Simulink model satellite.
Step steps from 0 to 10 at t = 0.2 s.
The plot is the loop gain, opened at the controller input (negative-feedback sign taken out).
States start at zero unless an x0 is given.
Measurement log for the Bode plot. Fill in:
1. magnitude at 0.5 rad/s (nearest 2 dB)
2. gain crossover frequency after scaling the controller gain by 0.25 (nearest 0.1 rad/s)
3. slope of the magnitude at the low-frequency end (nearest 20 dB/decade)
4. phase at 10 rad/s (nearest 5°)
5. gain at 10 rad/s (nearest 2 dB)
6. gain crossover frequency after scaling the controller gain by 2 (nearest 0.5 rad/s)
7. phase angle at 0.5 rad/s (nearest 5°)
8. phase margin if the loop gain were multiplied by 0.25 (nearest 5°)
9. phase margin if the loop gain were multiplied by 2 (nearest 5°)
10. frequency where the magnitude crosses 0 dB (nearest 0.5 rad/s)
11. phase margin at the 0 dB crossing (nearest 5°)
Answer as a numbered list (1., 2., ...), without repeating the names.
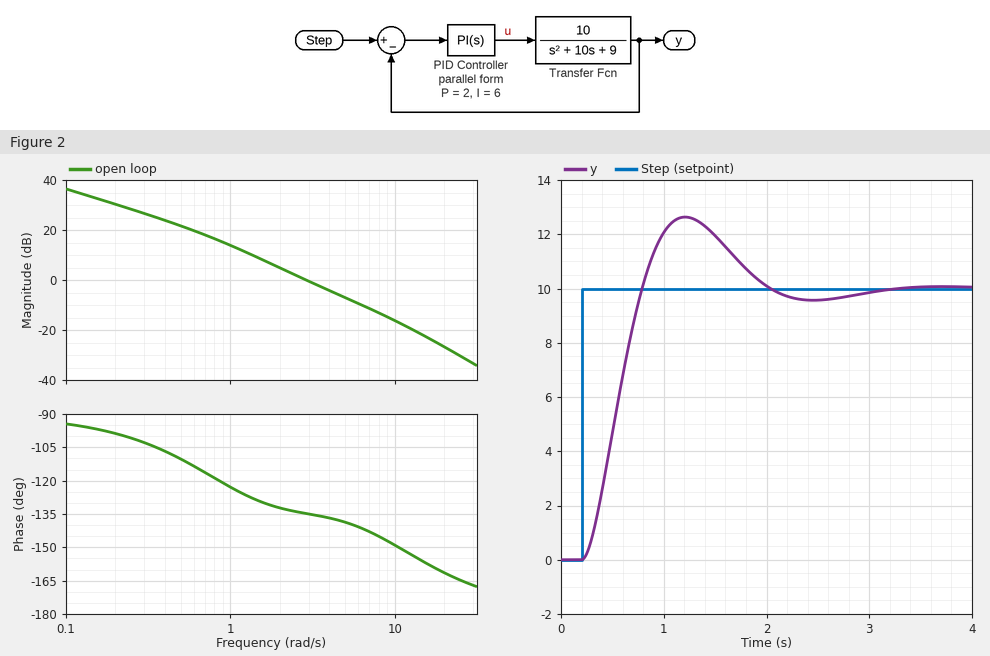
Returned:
1. 22 dB
2. 1.2 rad/s
3. -20 dB/decade
4. -150°
5. -16 dB
6. 4.5 rad/s
7. -110°
8. 55°
9. 40°
10. 3.0 rad/s
11. 45°
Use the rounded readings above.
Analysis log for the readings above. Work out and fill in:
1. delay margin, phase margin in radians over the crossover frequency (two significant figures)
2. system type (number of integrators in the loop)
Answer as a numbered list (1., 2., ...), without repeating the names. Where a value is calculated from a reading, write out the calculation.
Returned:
1. 45 × π / 180 / 3 = 0.26 s
2. 1
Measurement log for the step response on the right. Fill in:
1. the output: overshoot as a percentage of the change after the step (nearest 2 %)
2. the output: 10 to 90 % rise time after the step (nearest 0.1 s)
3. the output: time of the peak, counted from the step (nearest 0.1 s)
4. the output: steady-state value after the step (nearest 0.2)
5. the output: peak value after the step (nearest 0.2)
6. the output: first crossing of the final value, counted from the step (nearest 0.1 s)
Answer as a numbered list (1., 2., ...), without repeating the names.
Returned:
1. 26 %
2. 0.4 s
3. 1.0 s
4. 10.0
5. 12.6
6. 0.6 s
